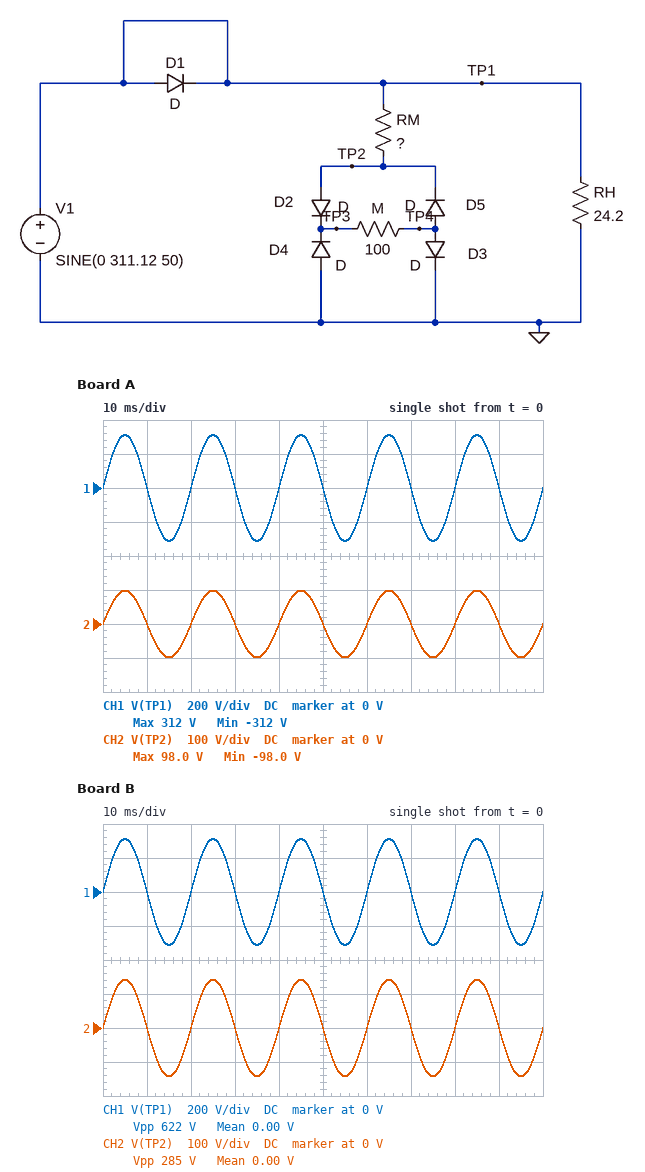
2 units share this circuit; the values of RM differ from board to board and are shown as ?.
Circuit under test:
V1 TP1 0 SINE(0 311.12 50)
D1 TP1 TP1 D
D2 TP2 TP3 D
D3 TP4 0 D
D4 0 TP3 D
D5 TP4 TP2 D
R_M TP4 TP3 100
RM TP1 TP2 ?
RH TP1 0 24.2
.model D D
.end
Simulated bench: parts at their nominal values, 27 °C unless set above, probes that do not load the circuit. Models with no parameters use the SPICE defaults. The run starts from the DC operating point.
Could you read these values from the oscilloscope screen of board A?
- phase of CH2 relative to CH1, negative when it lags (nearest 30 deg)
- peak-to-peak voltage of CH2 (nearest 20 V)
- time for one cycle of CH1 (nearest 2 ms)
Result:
0 deg
200 V
20 ms
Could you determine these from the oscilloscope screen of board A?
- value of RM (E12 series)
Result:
220 Ω
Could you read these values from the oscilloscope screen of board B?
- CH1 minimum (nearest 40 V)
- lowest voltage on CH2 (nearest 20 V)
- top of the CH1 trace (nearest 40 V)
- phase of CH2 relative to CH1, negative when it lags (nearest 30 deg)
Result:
-320 V
-140 V
320 V
0 deg
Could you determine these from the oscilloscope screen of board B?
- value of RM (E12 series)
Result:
120 Ω
